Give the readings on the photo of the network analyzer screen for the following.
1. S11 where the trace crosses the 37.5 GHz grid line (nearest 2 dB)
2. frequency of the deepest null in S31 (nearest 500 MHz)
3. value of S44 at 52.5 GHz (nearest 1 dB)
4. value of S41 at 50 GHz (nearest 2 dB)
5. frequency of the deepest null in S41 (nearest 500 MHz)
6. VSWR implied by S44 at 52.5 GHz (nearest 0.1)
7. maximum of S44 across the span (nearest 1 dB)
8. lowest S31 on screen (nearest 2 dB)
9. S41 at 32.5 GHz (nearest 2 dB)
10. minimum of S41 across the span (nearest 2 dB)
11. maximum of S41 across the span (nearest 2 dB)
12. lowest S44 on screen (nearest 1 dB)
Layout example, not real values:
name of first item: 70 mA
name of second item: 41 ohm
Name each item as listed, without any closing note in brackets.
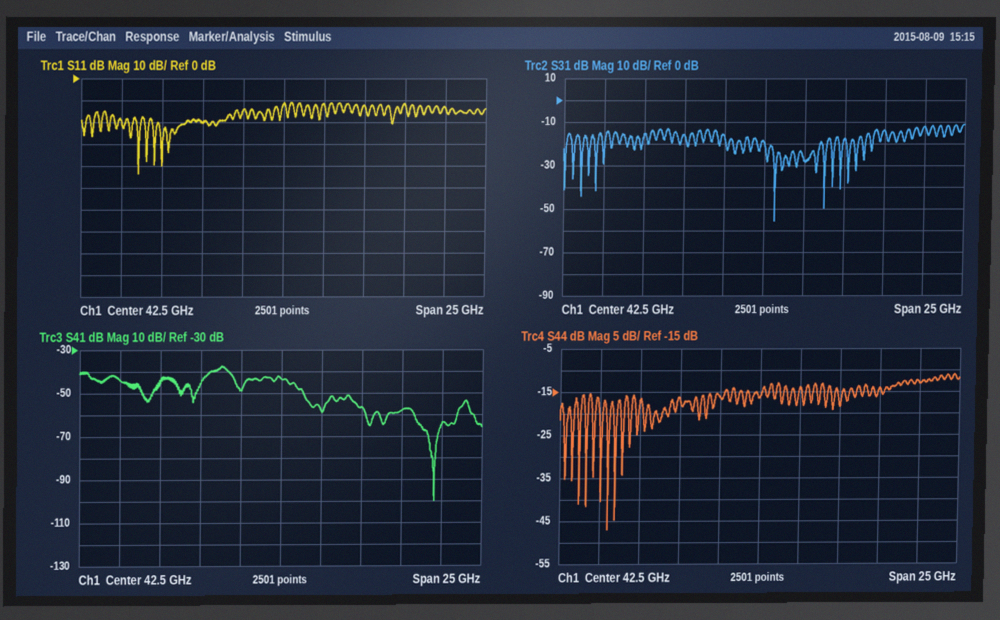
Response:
S11 where the trace crosses the 37.5 GHz grid line: -20 dB
frequency of the deepest null in S31: 43.0 GHz
value of S44 at 52.5 GHz: -13 dB
value of S41 at 50 GHz: -58 dB
frequency of the deepest null in S41: 52.0 GHz
VSWR implied by S44 at 52.5 GHz: 1.6
maximum of S44 across the span: -11 dB
lowest S31 on screen: -56 dB
S41 at 32.5 GHz: -44 dB
minimum of S41 across the span: -100 dB
maximum of S41 across the span: -38 dB
lowest S44 on screen: -47 dB
